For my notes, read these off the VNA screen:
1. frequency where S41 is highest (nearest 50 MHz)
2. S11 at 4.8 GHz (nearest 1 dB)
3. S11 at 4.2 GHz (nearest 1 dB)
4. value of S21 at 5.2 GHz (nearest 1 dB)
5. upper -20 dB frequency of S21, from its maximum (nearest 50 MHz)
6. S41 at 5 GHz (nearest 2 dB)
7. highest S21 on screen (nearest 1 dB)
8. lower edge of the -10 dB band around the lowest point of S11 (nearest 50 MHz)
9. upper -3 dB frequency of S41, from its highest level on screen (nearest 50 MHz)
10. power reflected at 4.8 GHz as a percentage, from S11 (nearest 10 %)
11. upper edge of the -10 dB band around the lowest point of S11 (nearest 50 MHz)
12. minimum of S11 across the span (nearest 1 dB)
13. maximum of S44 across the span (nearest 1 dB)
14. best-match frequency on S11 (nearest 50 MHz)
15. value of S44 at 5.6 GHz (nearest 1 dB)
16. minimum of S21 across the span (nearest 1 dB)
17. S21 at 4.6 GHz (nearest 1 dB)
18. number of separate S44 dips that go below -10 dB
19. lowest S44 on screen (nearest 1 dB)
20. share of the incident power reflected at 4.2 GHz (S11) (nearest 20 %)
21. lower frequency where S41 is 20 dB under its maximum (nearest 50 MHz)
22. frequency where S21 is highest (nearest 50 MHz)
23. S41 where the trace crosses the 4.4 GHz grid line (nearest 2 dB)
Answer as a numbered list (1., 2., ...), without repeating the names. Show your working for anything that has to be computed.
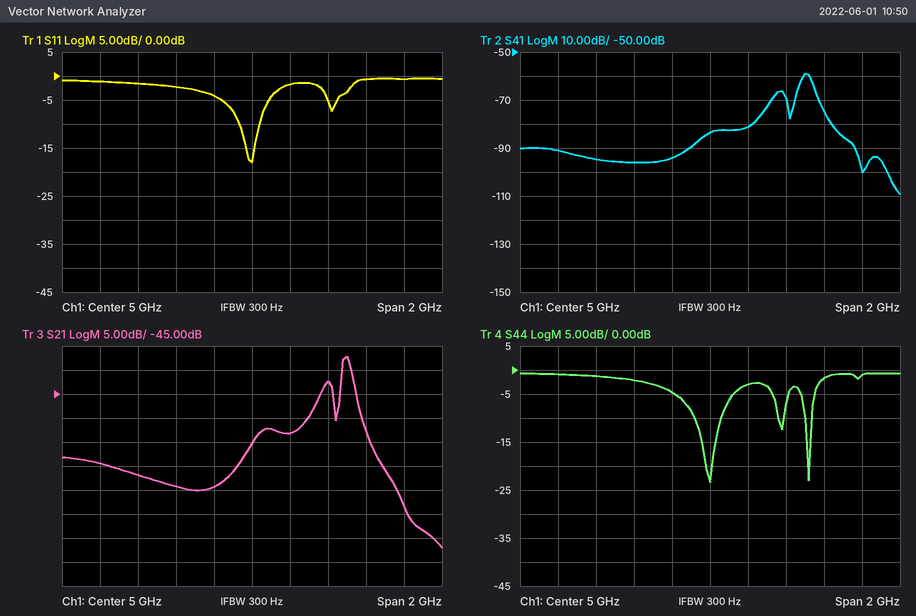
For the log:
1. 5.50 GHz
2. -4 dB
3. -1 dB
4. -53 dB
5. 5.65 GHz
6. -84 dB
7. -37 dB
8. 4.95 GHz
9. 5.55 GHz
10. 10^(-4/10) ≈ 40 %
11. 5.05 GHz
12. -18 dB
13. -1 dB
14. 5.00 GHz
15. -2 dB
16. -77 dB
17. -64 dB
18. 3
19. -23 dB
20. 10^(-1/10) ≈ 79.4 %, so 80 % to the nearest 20 %
21. 5.25 GHz
22. 5.50 GHz
23. -94 dB
